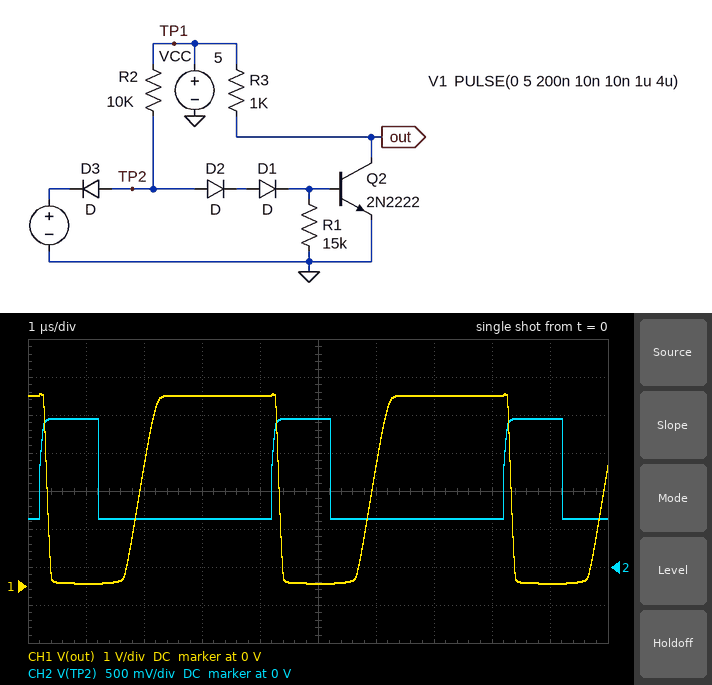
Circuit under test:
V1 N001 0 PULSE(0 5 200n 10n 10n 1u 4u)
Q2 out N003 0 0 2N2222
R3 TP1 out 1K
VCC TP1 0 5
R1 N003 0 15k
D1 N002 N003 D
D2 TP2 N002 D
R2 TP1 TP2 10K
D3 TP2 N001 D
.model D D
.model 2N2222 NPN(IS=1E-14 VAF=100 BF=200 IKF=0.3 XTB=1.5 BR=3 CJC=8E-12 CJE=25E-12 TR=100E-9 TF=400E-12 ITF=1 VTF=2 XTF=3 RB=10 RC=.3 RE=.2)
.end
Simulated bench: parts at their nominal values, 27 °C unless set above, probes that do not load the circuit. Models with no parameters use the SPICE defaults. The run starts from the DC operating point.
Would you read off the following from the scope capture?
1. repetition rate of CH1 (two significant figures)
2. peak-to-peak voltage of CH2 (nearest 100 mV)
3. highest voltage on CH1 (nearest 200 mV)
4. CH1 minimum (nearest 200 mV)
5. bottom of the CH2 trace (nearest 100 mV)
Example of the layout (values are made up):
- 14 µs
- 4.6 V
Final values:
- 250 kHz
- 1.3 V
- 5.0 V
- 0 V
- 600 mV
